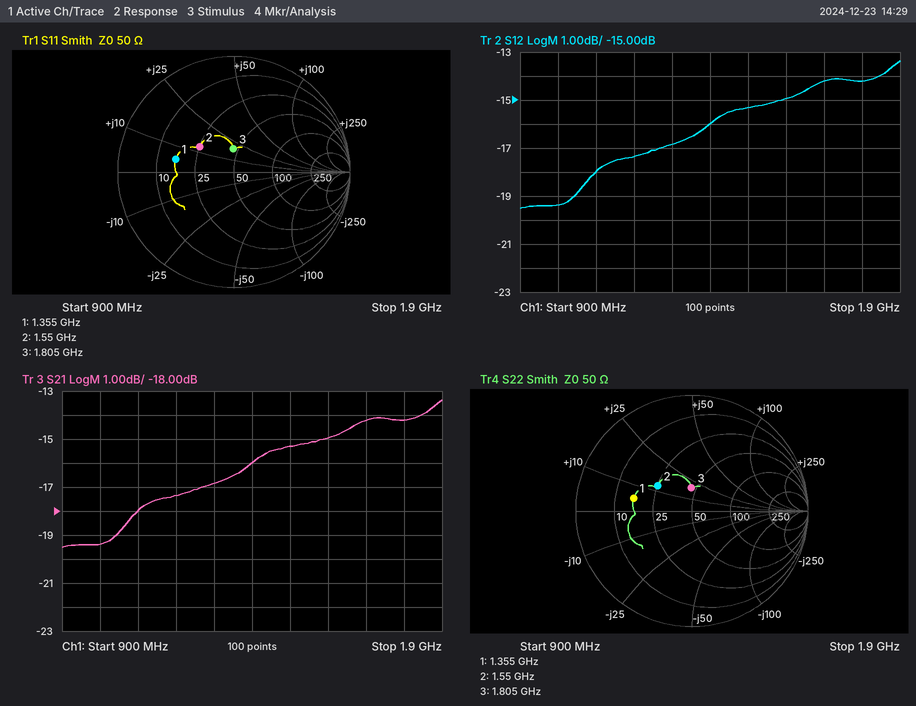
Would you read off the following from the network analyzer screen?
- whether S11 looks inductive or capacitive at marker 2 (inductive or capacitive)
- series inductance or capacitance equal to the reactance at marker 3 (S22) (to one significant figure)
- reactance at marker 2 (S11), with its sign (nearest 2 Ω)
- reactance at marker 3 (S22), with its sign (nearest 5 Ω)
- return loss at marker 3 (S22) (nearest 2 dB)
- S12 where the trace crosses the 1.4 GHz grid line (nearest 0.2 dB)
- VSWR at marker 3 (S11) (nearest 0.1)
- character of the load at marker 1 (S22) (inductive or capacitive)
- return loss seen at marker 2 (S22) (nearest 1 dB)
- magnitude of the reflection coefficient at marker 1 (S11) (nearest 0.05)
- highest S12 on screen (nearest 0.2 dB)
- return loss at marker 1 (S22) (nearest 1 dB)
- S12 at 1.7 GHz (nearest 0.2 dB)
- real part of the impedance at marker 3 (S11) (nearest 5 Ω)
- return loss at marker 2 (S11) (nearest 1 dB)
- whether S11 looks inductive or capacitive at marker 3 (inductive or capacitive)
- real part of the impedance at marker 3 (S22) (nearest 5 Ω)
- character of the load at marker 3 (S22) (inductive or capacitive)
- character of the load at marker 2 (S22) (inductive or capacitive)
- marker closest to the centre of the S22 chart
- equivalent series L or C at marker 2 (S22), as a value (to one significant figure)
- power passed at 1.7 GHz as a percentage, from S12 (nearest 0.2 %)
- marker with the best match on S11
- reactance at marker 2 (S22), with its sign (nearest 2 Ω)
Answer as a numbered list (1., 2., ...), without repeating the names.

1. inductive
2. 2 nH
3. +12 Ω
4. +20 Ω
5. 14 dB
6. -16.0 dB
7. 1.5
8. inductive
9. 9 dB
10. 0.50
11. -13.4 dB
12. 6 dB
13. -14.2 dB
14. 45 Ω
15. 9 dB
16. inductive
17. 45 Ω
18. inductive
19. inductive
20. marker 3
21. 1 nH
22. 3.8 %
23. marker 3
24. +12 Ω
